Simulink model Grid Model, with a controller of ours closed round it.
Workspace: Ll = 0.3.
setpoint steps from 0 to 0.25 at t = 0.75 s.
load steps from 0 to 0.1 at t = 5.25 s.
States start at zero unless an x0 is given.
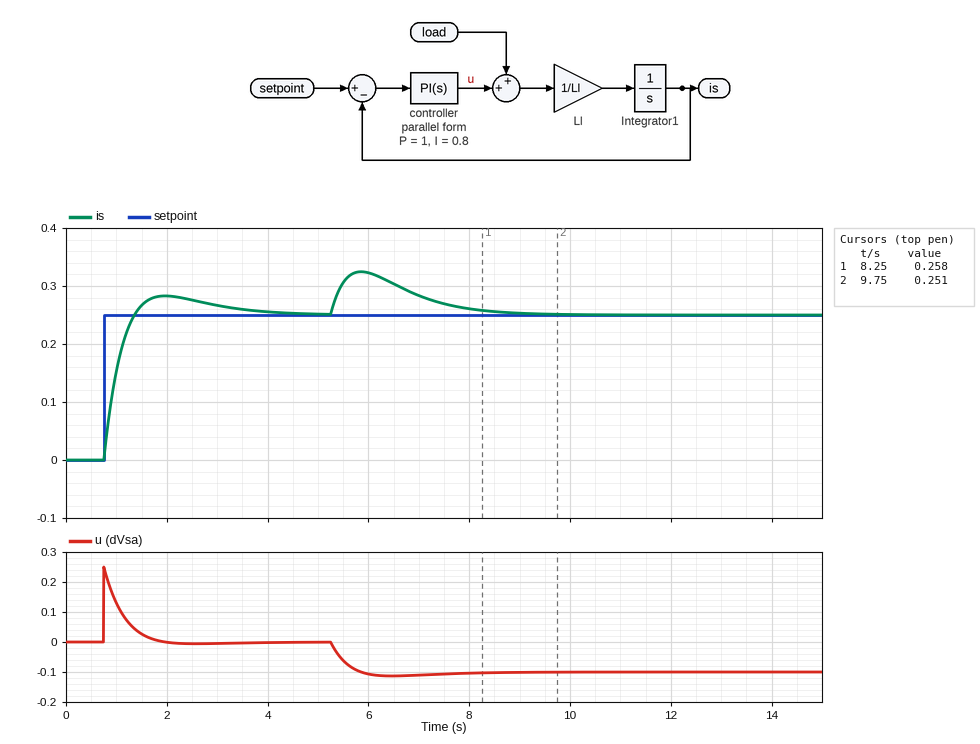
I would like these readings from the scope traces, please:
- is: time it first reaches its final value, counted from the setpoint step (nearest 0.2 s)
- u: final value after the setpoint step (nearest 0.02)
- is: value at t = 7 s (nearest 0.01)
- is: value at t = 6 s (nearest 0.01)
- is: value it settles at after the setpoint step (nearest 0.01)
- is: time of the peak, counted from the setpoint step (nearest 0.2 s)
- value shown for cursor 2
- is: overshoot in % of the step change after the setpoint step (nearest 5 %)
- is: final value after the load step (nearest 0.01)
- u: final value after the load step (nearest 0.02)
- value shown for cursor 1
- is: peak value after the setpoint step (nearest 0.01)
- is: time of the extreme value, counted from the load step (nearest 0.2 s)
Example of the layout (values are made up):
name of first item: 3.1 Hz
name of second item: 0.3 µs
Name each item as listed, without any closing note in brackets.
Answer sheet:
is: time it first reaches its final value, counted from the setpoint step: 0.6 s
u: final value after the setpoint step: 0.00
is: value at t = 7 s: 0.28
is: value at t = 6 s: 0.32
is: value it settles at after the setpoint step: 0.25
is: time of the peak, counted from the setpoint step: 1.2 s
value shown for cursor 2: 0.251
is: overshoot in % of the step change after the setpoint step: 15 %
is: final value after the load step: 0.25
u: final value after the load step: -0.10
value shown for cursor 1: 0.258
is: peak value after the setpoint step: 0.28
is: time of the extreme value, counted from the load step: 0.6 s
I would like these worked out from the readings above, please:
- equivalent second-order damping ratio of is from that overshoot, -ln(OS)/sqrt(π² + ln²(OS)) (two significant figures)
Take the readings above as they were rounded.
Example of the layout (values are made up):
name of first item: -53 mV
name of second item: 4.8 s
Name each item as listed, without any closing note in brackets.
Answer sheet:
equivalent second-order damping ratio of is from that overshoot, -ln(OS)/sqrt(π² + ln²(OS)): 0.52
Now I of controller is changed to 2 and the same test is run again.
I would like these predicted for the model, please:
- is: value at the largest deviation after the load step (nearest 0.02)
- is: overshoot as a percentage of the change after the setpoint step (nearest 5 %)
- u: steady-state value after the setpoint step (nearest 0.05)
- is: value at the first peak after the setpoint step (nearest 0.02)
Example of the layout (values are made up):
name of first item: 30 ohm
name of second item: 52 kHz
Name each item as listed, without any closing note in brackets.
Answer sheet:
is: value at the largest deviation after the load step: 0.32
is: overshoot as a percentage of the change after the setpoint step: 25 %
u: steady-state value after the setpoint step: 0.00
is: value at the first peak after the setpoint step: 0.30
